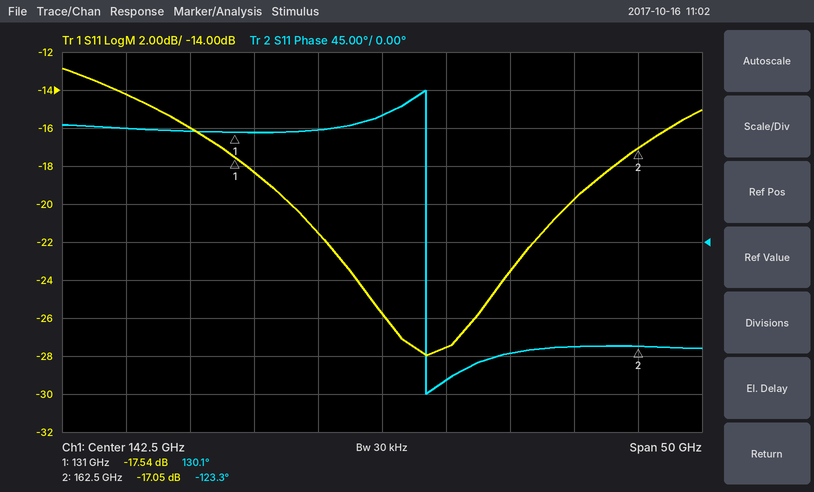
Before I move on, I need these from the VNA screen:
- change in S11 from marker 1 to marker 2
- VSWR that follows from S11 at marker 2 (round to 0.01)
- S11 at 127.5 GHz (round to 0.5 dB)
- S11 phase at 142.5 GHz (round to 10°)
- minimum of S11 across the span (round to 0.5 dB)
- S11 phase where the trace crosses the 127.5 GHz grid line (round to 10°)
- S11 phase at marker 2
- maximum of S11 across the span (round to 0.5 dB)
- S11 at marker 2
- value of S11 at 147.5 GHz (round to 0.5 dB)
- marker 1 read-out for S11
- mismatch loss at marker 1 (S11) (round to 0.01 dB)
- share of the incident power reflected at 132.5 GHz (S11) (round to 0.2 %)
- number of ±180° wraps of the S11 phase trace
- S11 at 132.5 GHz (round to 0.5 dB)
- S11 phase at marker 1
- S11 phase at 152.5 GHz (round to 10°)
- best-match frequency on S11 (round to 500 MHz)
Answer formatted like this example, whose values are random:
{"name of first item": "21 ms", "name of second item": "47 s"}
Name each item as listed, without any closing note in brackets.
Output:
{"change in S11 from marker 1 to marker 2": "0.49 dB", "VSWR that follows from S11 at marker 2": "1.33", "S11 at 127.5 GHz": "-16.0 dB", "S11 phase at 142.5 GHz": "150°", "minimum of S11 across the span": "-28.0 dB", "S11 phase where the trace crosses the 127.5 GHz grid line": "130°", "S11 phase at marker 2": "-123.3°", "maximum of S11 across the span": "-13.0 dB", "S11 at marker 2": "-17.05 dB", "value of S11 at 147.5 GHz": "-27.5 dB", "marker 1 read-out for S11": "-17.54 dB", "mismatch loss at marker 1 (S11)": "0.08 dB", "share of the incident power reflected at 132.5 GHz (S11)": "1.4 %", "number of ±180° wraps of the S11 phase trace": "1", "S11 at 132.5 GHz": "-18.5 dB", "S11 phase at marker 1": "130.1°", "S11 phase at 152.5 GHz": "-130°", "best-match frequency on S11": "146.0 GHz"}
